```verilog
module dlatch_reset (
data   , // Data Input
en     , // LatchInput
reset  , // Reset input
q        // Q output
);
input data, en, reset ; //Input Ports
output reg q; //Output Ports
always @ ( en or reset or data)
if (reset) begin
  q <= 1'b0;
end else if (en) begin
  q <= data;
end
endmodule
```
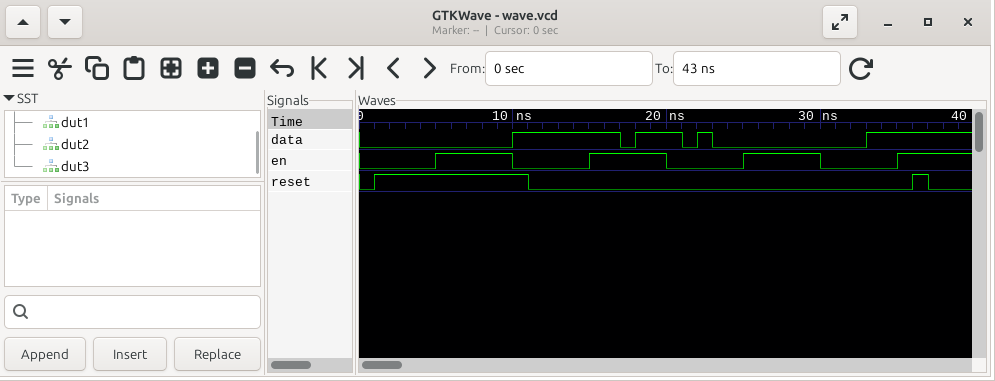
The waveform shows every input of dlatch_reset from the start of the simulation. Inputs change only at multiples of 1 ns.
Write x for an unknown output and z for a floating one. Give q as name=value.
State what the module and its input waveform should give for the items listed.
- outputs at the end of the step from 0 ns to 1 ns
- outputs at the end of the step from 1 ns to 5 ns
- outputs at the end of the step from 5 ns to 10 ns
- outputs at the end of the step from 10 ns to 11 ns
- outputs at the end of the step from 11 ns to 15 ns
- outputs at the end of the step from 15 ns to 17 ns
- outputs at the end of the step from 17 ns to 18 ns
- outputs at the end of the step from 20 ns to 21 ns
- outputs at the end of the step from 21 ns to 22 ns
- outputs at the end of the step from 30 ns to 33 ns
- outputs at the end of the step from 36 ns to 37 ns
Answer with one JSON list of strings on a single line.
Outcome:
["q=x", "q=0", "q=0", "q=0", "q=0", "q=1", "q=0", "q=1", "q=1", "q=0", "q=0"]
